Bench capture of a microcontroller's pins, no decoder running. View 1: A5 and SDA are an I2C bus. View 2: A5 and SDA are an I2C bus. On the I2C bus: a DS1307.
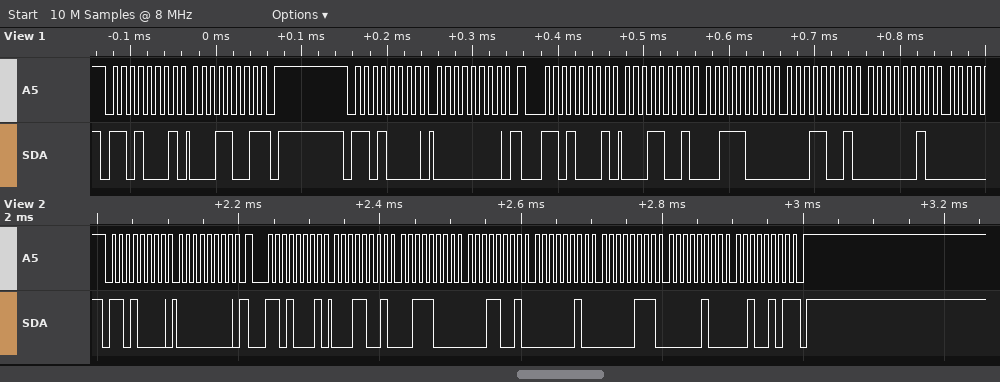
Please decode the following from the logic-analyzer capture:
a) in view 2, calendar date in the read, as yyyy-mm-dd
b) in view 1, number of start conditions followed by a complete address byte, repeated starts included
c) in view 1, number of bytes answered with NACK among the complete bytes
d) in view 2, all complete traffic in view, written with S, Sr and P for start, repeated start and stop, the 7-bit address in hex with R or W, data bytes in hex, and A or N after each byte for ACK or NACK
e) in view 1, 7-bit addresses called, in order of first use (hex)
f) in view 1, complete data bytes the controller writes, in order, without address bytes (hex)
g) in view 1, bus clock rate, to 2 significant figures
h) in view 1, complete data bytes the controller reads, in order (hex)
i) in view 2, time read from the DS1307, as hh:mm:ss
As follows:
2025-04-07
3
1
S 68W A 00 A Sr 68R A 19 A 38 A 19 A 02 A 07 A 04 A 25 N P
0x68
00
100 kHz
19 19 38 19 02
19:38:19
